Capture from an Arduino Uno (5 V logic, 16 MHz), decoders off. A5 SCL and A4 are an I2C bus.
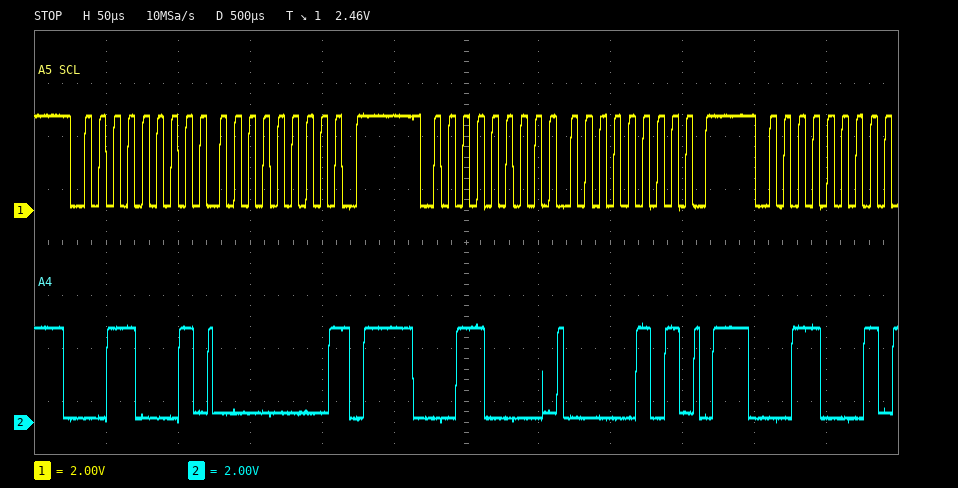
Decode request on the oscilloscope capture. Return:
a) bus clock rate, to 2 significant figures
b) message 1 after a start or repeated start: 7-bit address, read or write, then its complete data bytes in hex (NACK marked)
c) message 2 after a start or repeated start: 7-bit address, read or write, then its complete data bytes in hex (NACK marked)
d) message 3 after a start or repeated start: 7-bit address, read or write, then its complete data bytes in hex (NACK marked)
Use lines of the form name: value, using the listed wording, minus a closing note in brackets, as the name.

bus clock rate, to 2 significant figures: 100 kHz
message 1 after a start or repeated start: 7-bit address, read or write, then its complete data bytes in hex: 0x18 read: 00 NACK
message 2 after a start or repeated start: 7-bit address, read or write, then its complete data bytes in hex: 0x18 write: 05
message 3 after a start or repeated start: 7-bit address, read or write, then its complete data bytes in hex: 0x18 read
